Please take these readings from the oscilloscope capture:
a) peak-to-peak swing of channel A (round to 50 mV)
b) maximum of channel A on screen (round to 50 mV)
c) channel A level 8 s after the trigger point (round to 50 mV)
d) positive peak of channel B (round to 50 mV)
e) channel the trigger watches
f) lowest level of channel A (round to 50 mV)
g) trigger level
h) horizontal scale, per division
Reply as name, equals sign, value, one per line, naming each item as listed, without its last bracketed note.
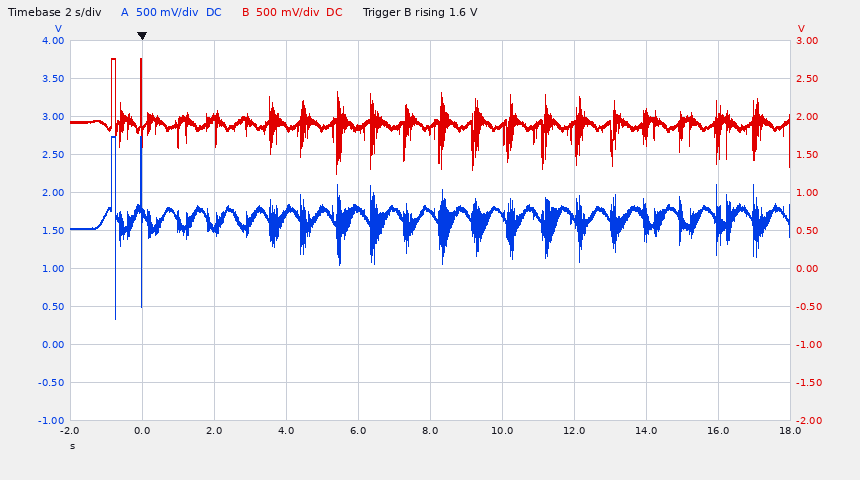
peak-to-peak swing of channel A = 2.40 V
maximum of channel A on screen = 2.75 V
channel A level 8 s after the trigger point = 1.75 V
positive peak of channel B = 2.75 V
channel the trigger watches = channel B
lowest level of channel A = 350 mV
trigger level = 1.6 V
horizontal scale, per division = 2 s
